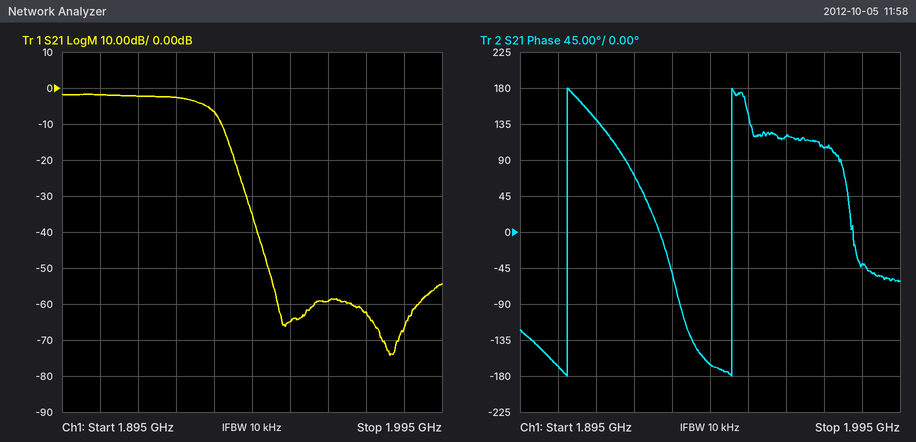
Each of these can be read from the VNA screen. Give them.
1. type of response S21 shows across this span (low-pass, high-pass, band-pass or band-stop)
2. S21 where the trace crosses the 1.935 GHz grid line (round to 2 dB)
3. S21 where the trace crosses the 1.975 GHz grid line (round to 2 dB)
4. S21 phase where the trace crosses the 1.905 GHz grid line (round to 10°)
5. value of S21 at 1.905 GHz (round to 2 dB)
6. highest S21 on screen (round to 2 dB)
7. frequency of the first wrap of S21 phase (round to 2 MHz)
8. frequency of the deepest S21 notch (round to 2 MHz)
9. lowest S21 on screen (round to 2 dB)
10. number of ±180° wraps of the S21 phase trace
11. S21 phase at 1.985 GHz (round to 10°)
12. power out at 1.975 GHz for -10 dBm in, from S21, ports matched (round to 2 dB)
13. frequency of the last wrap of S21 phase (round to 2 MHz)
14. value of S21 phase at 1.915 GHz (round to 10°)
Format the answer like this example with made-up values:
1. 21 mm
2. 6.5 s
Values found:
1. low-pass
2. -6 dB
3. -62 dB
4. -170°
5. -2 dB
6. -2 dB
7. 1.908 GHz
8. 1.982 GHz
9. -74 dB
10. 2
11. -40°
12. -72 dBm
13. 1.950 GHz
14. 140°
